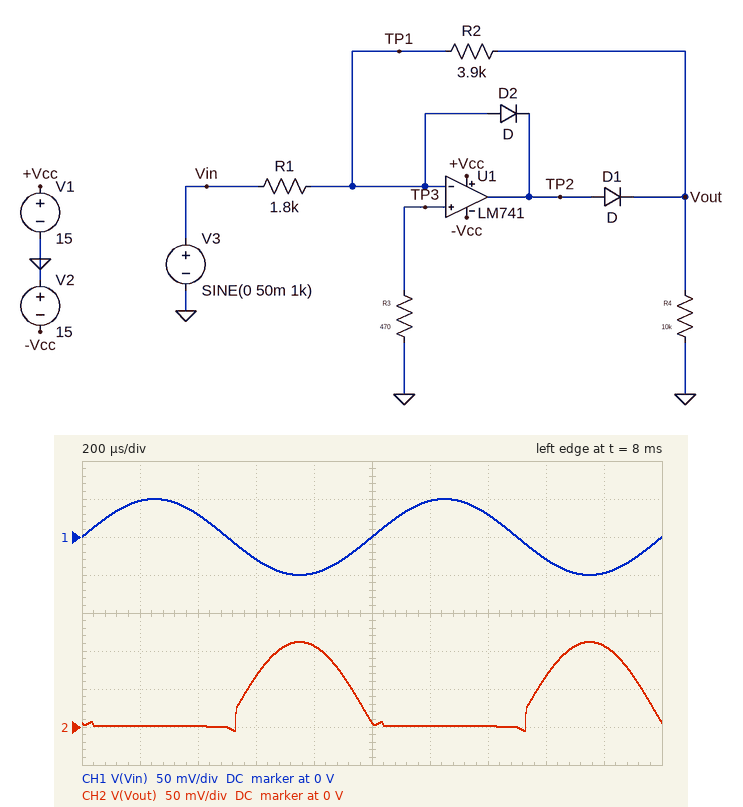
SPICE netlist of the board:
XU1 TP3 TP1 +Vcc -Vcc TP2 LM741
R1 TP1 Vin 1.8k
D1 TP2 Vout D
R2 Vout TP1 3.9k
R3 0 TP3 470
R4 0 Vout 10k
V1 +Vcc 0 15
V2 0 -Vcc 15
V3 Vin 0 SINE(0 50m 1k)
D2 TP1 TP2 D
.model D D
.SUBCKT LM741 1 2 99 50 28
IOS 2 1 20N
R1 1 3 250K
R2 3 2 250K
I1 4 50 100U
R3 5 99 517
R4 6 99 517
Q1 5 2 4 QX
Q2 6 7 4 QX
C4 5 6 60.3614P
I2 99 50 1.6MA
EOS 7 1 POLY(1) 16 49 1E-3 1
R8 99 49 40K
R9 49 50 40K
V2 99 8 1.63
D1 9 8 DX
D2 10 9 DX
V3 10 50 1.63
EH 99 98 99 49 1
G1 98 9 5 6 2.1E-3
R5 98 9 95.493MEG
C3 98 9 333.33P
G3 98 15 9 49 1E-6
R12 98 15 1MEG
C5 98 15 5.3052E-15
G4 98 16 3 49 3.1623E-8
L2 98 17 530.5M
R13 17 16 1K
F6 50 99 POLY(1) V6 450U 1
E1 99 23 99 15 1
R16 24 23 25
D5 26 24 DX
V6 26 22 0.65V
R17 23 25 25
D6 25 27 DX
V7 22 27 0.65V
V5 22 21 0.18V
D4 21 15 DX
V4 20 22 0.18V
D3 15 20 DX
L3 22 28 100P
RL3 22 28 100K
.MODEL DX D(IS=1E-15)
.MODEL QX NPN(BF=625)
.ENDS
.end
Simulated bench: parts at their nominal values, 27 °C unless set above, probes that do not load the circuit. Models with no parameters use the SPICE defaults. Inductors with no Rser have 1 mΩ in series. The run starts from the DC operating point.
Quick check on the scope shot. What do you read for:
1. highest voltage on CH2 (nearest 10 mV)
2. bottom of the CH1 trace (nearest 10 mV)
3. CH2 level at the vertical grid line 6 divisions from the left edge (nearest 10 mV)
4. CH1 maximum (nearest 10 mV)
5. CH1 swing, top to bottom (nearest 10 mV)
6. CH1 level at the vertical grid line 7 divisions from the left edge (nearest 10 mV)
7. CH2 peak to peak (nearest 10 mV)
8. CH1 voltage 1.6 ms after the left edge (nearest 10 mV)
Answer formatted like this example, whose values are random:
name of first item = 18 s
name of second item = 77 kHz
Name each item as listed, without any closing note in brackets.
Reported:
highest voltage on CH2 = 110 mV
bottom of the CH1 trace = -50 mV
CH2 level at the vertical grid line 6 divisions from the left edge = 0 V
CH1 maximum = 50 mV
CH1 swing, top to bottom = 100 mV
CH1 level at the vertical grid line 7 divisions from the left edge = 30 mV
CH2 peak to peak = 120 mV
CH1 voltage 1.6 ms after the left edge = -30 mV
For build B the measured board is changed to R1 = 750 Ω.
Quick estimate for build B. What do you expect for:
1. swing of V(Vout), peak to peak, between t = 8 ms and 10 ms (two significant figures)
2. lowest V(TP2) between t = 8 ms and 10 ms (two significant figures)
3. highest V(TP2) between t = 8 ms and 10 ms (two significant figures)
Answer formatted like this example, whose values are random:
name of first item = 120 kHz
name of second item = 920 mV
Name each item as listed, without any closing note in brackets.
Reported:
swing of V(Vout), peak to peak, between t = 8 ms and 10 ms = 270 mV
lowest V(TP2) between t = 8 ms and 10 ms = -580 mV
highest V(TP2) between t = 8 ms and 10 ms = 860 mV
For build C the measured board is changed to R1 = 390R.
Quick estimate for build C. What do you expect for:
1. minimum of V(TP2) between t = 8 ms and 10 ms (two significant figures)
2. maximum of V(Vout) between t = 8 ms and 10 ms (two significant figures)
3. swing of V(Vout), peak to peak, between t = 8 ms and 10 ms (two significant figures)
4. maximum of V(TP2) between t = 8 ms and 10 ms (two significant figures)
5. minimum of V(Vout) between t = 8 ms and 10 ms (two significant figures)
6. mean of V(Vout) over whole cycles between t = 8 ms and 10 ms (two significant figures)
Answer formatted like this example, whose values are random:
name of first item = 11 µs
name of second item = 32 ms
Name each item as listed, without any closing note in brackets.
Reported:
minimum of V(TP2) between t = 8 ms and 10 ms = -600 mV
maximum of V(Vout) between t = 8 ms and 10 ms = 510 mV
swing of V(Vout), peak to peak, between t = 8 ms and 10 ms = 520 mV
maximum of V(TP2) between t = 8 ms and 10 ms = 1.1 V
minimum of V(Vout) between t = 8 ms and 10 ms = -5.8 mV
mean of V(Vout) over whole cycles between t = 8 ms and 10 ms = 160 mV
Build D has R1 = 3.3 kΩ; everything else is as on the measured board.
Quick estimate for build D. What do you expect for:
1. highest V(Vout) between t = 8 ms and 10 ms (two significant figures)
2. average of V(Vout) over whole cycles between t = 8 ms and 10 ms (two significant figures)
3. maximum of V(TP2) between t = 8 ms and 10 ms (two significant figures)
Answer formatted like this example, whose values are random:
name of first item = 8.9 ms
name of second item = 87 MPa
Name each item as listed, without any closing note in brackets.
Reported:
highest V(Vout) between t = 8 ms and 10 ms = 62 mV
average of V(Vout) over whole cycles between t = 8 ms and 10 ms = 20 mV
maximum of V(TP2) between t = 8 ms and 10 ms = 620 mV
